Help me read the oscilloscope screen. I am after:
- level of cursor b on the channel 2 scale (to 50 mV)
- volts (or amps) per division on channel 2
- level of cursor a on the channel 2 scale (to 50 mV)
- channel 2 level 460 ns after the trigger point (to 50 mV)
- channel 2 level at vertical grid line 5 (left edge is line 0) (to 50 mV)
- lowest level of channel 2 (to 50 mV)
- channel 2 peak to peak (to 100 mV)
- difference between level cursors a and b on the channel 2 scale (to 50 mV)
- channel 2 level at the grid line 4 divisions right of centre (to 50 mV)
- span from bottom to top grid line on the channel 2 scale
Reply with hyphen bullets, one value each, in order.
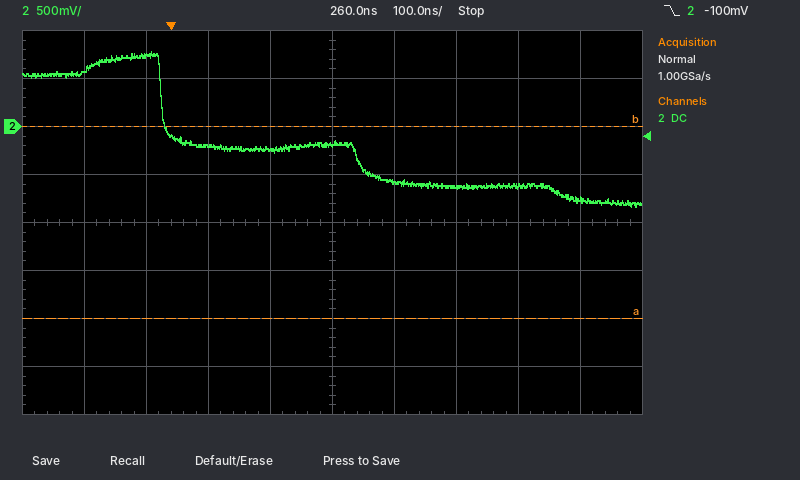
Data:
- 0 mV
- 500 mV
- -2.00 V
- -650 mV
- -200 mV
- -850 mV
- 1.60 V
- 2.00 V
- -750 mV
- 4 V
